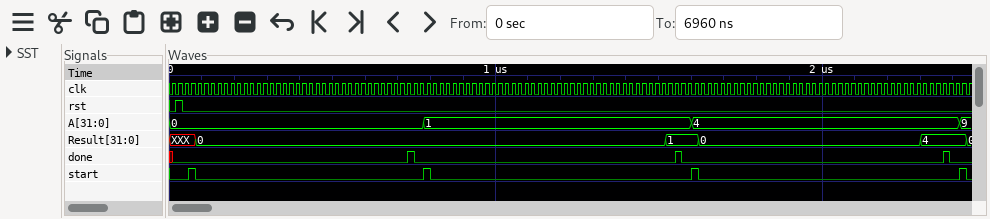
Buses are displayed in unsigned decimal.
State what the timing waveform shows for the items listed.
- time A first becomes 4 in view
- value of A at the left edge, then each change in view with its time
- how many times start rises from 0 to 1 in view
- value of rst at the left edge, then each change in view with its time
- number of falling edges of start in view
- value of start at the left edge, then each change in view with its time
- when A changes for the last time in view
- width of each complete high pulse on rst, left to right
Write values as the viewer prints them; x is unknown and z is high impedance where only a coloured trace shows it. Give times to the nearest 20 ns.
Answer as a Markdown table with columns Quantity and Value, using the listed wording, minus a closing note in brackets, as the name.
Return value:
| Quantity | Value |
|---|---|
| time A first becomes 4 in view | 1600 ns |
| value of A at the left edge, then each change in view with its time | 0, 1 at 780 ns, 4 at 1600 ns, 9 at 2420 ns |
| how many times start rises from 0 to 1 in view | 4 |
| value of rst at the left edge, then each change in view with its time | 0, 1 at 20 ns, 0 at 40 ns |
| number of falling edges of start in view | 4 |
| value of start at the left edge, then each change in view with its time | 0, 1 at 60 ns, 0 at 80 ns, 1 at 780 ns, 0 at 800 ns, 1 at 1600 ns, 0 at 1620 ns, 1 at 2420 ns, 0 at 2440 ns |
| when A changes for the last time in view | 2420 ns |
| width of each complete high pulse on rst, left to right | 20 ns |
